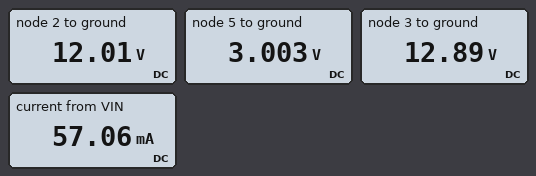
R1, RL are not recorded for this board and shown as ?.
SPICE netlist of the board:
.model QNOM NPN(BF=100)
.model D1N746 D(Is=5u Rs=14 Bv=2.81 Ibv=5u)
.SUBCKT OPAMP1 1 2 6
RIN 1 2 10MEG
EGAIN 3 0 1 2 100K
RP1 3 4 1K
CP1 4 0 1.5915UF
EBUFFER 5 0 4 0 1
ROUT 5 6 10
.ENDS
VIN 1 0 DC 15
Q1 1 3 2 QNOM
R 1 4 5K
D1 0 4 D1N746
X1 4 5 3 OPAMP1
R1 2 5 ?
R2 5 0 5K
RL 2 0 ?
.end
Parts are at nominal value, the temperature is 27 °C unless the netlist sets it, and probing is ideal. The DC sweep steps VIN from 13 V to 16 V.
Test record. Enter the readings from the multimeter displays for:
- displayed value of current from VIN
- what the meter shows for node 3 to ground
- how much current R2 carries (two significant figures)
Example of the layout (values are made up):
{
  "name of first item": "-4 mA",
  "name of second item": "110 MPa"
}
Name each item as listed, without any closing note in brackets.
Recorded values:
{
  "displayed value of current from VIN": "57.06 mA",
  "what the meter shows for node 3 to ground": "12.89 V",
  "how much current R2 carries": "600 µA"
}
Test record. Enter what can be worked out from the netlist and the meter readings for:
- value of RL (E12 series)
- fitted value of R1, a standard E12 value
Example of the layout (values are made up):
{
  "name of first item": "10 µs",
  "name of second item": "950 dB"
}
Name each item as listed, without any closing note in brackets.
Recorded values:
{
  "value of RL": "220 Ω",
  "fitted value of R1, a standard E12 value": "15 kΩ"
}
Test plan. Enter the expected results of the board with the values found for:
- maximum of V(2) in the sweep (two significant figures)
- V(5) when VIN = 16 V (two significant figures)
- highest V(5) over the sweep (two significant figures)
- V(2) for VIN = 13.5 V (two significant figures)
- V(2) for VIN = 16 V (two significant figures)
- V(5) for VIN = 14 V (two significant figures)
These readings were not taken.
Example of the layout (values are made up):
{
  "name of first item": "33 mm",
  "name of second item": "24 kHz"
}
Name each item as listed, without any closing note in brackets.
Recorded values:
{
  "maximum of V(2) in the sweep": "12 V",
  "V(5) when VIN = 16 V": "3.0 V",
  "highest V(5) over the sweep": "3.0 V",
  "V(2) for VIN = 13.5 V": "12 V",
  "V(2) for VIN = 16 V": "12 V",
  "V(5) for VIN = 14 V": "3.0 V"
}
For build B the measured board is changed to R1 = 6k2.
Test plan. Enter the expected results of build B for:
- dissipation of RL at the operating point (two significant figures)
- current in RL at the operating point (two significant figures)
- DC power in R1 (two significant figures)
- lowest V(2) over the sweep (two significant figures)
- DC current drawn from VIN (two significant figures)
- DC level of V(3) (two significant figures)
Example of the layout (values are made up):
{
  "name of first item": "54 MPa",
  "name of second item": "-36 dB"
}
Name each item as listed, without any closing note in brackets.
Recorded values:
{
  "dissipation of RL at the operating point": "210 mW",
  "current in RL at the operating point": "31 mA",
  "DC power in R1": "2.2 mW",
  "lowest V(2) over the sweep": "6.7 V",
  "DC current drawn from VIN": "33 mA",
  "DC level of V(3)": "7.6 V"
}
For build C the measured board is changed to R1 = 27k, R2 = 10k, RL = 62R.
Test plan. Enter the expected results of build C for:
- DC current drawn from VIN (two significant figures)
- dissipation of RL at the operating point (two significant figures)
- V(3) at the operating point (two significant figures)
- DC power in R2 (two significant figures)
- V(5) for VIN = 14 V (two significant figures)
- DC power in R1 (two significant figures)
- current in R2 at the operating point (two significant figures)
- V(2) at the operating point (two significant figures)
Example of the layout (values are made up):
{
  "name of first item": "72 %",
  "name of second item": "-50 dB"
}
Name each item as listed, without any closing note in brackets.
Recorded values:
{
  "DC current drawn from VIN": "180 mA",
  "dissipation of RL at the operating point": "2.0 W",
  "V(3) at the operating point": "12 V",
  "DC power in R2": "900 µW",
  "V(5) for VIN = 14 V": "3.0 V",
  "DC power in R1": "2.4 mW",
  "current in R2 at the operating point": "300 µA",
  "V(2) at the operating point": "11 V"
}
